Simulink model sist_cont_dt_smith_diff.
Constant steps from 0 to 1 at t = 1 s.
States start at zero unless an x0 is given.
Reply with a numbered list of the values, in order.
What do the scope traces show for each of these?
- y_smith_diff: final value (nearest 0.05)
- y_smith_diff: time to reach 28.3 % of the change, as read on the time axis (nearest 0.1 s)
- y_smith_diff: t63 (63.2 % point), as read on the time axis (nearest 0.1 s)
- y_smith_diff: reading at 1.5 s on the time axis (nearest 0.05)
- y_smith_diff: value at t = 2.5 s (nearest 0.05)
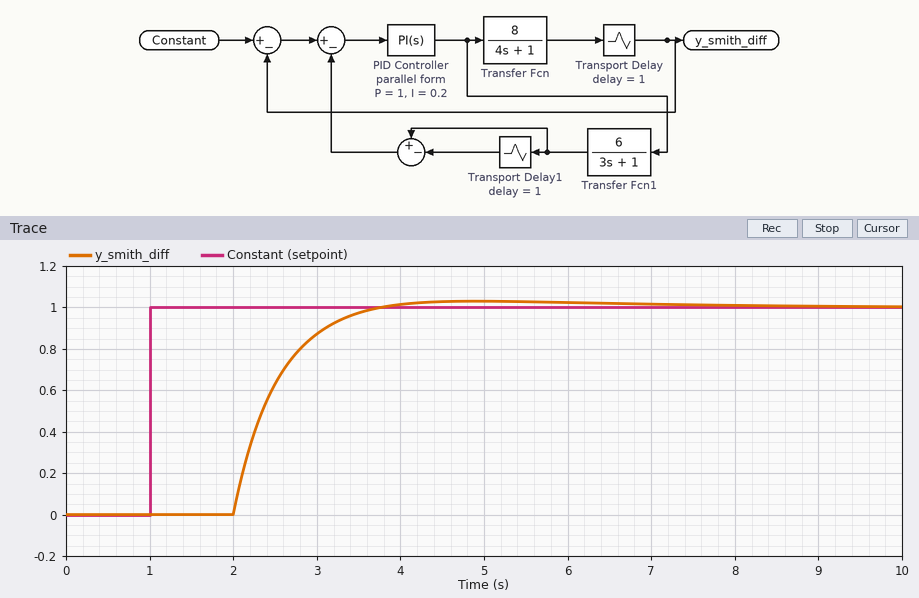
1. 1.00
2. 2.2 s
3. 2.5 s
4. 0.00
5. 0.65
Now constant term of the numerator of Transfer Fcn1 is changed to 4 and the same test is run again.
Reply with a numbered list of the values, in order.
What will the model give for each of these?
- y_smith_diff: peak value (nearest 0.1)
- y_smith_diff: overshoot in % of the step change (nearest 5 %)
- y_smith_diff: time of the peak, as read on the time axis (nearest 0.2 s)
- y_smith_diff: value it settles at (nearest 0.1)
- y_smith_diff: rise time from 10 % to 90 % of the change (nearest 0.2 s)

1. 1.2
2. 20 %
3. 3.4 s
4. 1.0
5. 0.6 s
